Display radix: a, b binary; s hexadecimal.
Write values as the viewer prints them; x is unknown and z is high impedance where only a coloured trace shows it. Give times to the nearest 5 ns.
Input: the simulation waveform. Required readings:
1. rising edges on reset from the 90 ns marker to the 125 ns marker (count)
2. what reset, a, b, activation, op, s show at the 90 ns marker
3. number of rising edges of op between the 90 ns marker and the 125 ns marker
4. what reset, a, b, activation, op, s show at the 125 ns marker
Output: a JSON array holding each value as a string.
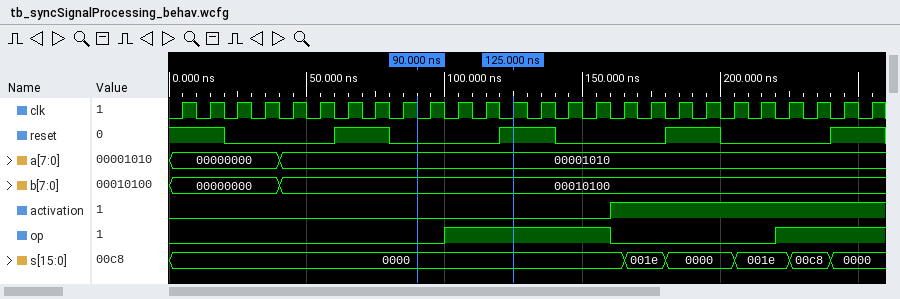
["1", "reset=0, a=00001010, b=00010100, activation=0, op=0, s=0000", "1", "reset=1, a=00001010, b=00010100, activation=0, op=1, s=0000"]
